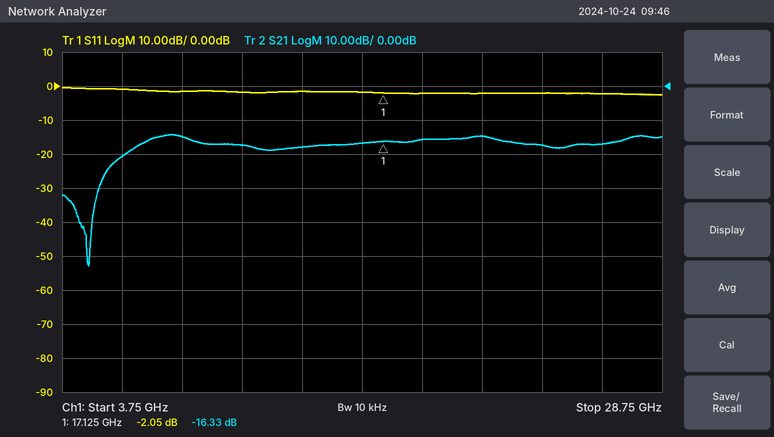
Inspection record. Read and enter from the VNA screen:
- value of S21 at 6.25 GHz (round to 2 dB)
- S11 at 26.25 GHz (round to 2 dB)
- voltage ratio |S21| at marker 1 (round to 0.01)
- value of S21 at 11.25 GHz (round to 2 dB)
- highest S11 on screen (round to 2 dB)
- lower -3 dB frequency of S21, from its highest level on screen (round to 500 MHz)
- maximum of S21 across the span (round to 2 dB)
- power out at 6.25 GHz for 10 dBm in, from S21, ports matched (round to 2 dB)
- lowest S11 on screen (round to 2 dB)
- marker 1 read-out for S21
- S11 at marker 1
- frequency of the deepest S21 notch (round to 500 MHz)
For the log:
-20 dB
-2 dB
0.15
-18 dB
0 dB
7.0 GHz
-14 dB
-10 dBm
-2 dB
-16.33 dB
-2.05 dB
5.0 GHz
